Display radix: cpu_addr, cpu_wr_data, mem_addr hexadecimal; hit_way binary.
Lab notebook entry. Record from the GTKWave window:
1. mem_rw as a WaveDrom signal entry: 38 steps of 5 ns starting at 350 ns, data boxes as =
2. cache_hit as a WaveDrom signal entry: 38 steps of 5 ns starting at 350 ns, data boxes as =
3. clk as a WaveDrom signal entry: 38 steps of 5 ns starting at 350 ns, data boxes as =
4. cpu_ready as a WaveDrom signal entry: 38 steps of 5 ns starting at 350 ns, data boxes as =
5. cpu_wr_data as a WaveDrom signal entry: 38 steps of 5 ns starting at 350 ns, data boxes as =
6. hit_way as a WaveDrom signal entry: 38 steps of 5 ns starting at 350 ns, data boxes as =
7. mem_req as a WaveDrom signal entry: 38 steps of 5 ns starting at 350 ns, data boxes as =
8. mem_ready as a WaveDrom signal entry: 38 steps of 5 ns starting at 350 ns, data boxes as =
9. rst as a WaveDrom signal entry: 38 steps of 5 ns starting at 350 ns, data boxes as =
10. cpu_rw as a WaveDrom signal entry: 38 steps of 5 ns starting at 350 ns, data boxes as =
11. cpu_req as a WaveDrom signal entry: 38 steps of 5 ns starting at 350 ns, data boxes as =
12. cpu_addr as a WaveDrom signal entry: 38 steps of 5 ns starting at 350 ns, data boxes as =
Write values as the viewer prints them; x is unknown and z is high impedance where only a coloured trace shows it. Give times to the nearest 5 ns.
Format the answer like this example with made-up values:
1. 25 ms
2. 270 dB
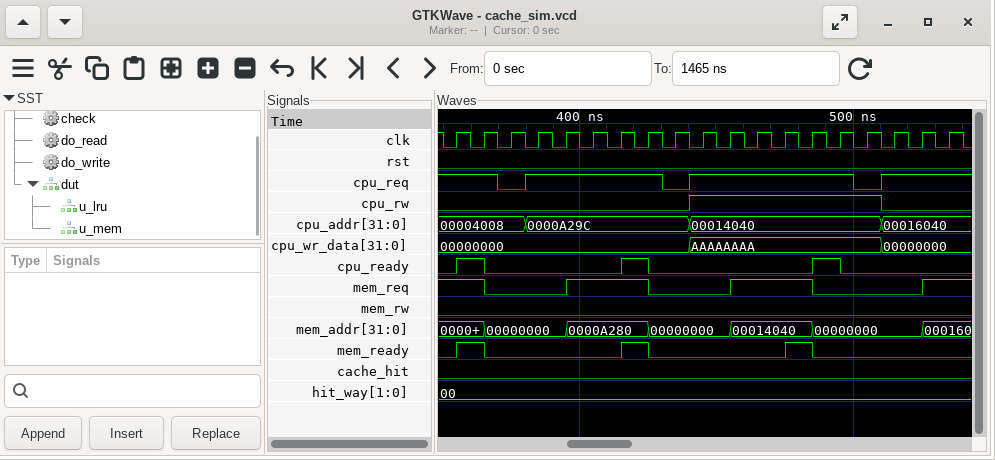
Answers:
1. {name: 'mem_rw', wave: '0.....................................'}
2. {name: 'cache_hit', wave: '0.....................................'}
3. {name: 'clk', wave: '01010101010101010101010101010101010101'}
4. {name: 'cpu_ready', wave: '01.0.........1.0...........1.0........'}
5. {name: 'cpu_wr_data', wave: '=.................=.............=.....', data: '00000000 AAAAAAAA 00000000'}
6. {name: 'hit_way', wave: '=.....................................', data: '00'}
7. {name: 'mem_req', wave: '1..0.....1.....0.....1.....0.......1..'}
8. {name: 'mem_ready', wave: '01.0.........1.0.........1.0..........'}
9. {name: 'rst', wave: '0.....................................'}
10. {name: 'cpu_rw', wave: '0.................1.............0.....'}
11. {name: 'cpu_req', wave: '1...0.1.........0.1...........0.1.....'}
12. {name: 'cpu_addr', wave: '=.....=...........=.............=.....', data: '00004008 0000A29C 00014040 00016040'}
